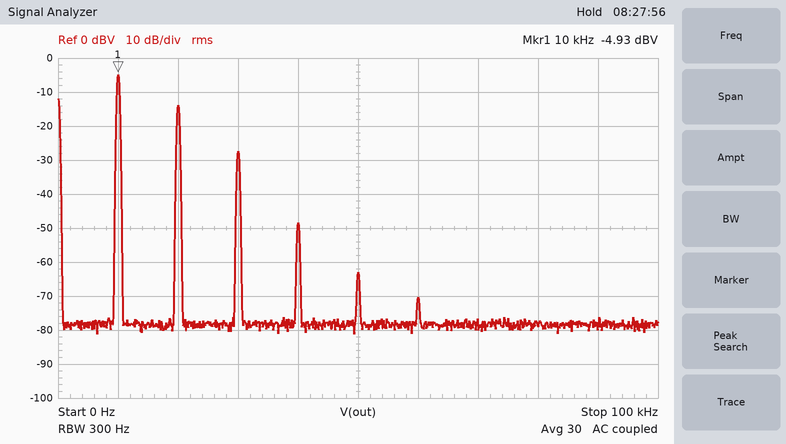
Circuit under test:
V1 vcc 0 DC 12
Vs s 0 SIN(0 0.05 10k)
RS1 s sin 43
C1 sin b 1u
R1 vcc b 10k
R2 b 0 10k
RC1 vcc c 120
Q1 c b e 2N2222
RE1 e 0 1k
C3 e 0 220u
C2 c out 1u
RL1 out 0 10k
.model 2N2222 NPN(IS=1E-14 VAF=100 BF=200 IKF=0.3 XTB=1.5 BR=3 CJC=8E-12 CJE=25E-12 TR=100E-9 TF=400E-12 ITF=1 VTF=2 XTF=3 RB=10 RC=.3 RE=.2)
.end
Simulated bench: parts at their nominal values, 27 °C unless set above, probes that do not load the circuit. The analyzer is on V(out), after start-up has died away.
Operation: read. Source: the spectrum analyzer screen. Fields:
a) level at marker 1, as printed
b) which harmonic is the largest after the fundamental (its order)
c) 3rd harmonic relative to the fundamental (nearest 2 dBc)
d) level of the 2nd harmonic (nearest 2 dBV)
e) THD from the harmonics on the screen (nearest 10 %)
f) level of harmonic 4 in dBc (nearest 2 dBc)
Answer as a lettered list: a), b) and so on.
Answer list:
a) -4.93 dBV
b) 2
c) -22 dBc
d) -14 dBV
e) 40 %
f) -44 dBc
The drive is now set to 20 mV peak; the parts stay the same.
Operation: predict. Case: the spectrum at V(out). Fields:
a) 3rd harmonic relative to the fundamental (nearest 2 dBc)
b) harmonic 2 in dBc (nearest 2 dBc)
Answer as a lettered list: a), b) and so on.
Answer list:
a) -38 dBc
b) -16 dBc
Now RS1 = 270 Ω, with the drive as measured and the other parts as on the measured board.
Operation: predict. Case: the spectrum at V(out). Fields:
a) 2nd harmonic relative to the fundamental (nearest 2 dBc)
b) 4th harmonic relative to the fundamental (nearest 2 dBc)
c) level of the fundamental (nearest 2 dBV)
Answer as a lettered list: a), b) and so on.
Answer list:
a) -12 dBc
b) -46 dBc
c) -6 dBV
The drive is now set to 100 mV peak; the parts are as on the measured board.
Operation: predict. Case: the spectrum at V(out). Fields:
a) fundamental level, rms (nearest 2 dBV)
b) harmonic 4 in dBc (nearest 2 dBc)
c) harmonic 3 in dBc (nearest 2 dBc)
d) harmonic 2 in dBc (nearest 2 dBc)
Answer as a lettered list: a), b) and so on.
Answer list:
a) -2 dBV
b) -24 dBc
c) -12 dBc
d) -4 dBc
